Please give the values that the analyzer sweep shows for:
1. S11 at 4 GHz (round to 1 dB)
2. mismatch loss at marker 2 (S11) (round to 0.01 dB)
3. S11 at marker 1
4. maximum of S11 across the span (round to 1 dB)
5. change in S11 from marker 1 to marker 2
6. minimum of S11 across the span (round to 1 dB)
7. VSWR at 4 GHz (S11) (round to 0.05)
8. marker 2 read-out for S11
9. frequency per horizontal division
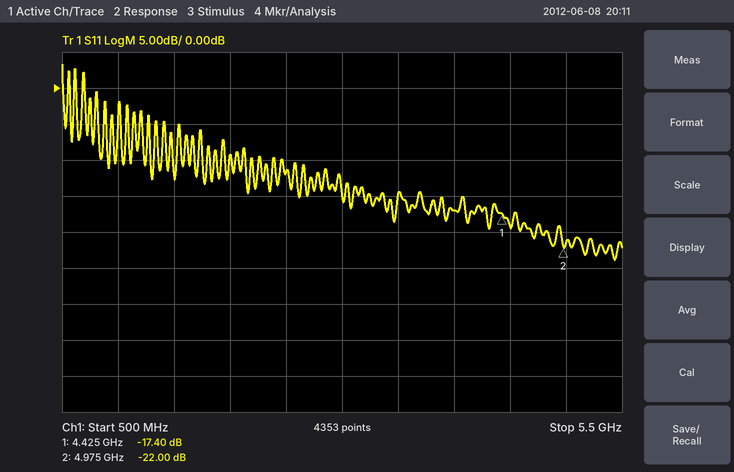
-17 dB
0.03 dB
-17.40 dB
3 dB
-4.60 dB
-24 dB
1.35
-22.00 dB
500 MHz
